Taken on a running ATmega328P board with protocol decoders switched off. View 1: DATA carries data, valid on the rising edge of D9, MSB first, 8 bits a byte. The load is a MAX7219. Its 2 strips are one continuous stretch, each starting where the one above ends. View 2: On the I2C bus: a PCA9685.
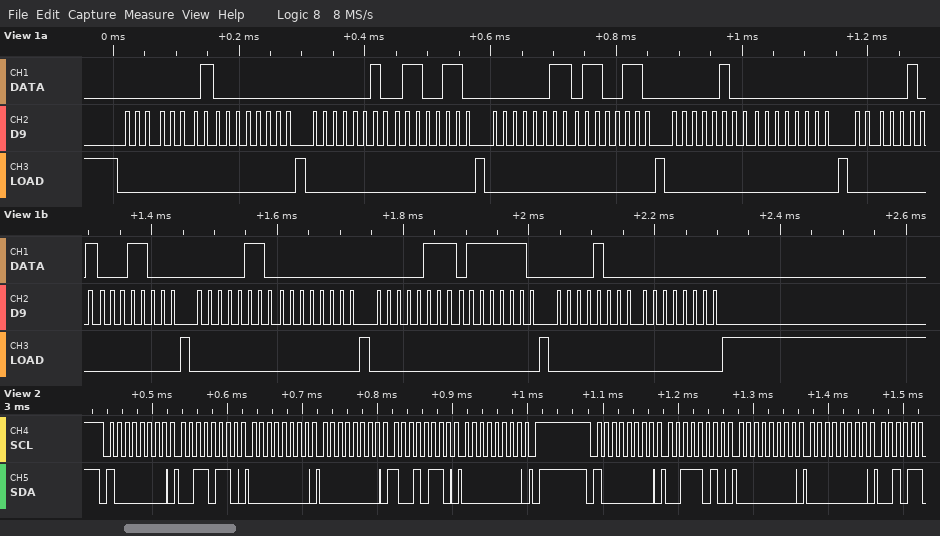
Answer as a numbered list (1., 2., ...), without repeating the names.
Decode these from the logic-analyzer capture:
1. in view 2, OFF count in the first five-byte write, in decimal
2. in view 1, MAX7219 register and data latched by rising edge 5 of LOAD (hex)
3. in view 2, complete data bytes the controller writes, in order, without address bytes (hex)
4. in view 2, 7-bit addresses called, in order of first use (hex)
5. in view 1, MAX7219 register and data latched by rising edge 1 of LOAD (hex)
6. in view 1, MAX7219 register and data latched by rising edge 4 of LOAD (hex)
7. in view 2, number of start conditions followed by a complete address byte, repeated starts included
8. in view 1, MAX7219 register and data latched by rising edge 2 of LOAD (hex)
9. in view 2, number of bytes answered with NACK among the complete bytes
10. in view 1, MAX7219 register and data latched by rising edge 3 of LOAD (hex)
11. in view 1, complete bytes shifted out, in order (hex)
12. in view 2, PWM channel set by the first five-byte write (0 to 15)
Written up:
1. 150
2. register 0x5, data 0x18
3. 36 00 00 96 00 3A 00 00
4. 0x40
5. register 0x1, data 0x00
6. register 0x4, data 0x00
7. 2
8. register 0x2, data 0x66
9. 0
10. register 0x3, data 0x66
11. 01 00 02 66 03 66 04 00 05 18 06 00 07 7E 08 00
12. 12
